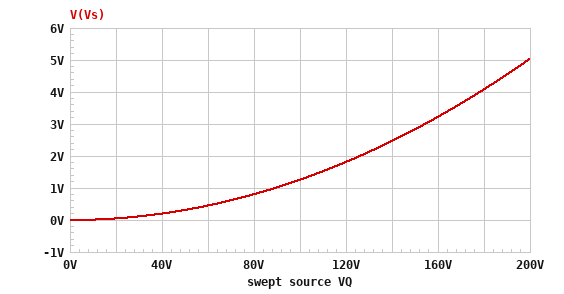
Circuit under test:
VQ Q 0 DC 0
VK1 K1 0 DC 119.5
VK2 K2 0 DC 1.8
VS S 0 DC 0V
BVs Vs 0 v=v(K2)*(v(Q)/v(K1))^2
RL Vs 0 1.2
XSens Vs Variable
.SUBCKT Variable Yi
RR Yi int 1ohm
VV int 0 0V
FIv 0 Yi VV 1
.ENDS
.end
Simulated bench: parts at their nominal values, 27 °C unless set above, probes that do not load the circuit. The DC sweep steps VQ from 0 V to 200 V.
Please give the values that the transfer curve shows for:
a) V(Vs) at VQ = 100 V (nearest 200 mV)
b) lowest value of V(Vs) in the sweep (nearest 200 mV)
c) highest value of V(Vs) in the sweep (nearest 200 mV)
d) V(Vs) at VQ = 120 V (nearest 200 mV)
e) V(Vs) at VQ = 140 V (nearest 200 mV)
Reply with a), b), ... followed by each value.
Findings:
a) 1.2 V
b) 0 V
c) 5.0 V
d) 1.8 V
e) 2.4 V
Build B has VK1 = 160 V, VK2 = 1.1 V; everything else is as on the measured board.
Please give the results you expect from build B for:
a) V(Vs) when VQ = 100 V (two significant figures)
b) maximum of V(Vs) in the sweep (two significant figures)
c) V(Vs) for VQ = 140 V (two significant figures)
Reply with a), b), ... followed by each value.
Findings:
a) 430 mV
b) 1.7 V
c) 840 mV
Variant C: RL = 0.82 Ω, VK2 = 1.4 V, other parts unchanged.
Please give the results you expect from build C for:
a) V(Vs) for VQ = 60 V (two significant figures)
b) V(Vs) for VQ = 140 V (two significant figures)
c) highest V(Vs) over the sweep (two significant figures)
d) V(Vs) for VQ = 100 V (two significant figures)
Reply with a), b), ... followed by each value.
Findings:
a) 350 mV
b) 1.9 V
c) 3.9 V
d) 980 mV
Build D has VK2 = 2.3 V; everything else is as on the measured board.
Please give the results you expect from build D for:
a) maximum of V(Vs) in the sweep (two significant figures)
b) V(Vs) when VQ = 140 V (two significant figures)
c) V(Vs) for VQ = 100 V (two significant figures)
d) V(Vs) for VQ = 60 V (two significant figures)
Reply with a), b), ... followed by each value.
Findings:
a) 6.4 V
b) 3.2 V
c) 1.6 V
d) 580 mV
